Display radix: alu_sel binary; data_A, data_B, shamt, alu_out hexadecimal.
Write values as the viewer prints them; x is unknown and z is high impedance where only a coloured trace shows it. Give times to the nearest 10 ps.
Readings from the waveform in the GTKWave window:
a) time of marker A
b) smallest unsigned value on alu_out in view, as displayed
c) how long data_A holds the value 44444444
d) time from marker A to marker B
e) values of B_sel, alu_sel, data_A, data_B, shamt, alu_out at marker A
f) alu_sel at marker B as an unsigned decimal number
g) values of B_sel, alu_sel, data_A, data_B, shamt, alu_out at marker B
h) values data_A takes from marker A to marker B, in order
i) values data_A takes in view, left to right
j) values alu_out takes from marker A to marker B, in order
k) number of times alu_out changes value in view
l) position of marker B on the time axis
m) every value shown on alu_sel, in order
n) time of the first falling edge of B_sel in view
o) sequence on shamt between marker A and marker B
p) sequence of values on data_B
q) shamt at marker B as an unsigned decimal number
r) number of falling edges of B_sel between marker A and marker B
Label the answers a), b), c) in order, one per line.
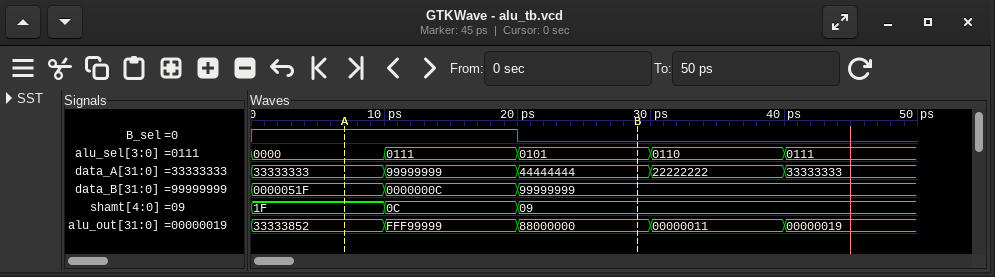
a) 10 ps
b) 00000011
c) 10 ps
d) 20 ps
e) B_sel=1, alu_sel=0000, data_A=33333333, data_B=0000051F, shamt=1F, alu_out=33333852
f) 5
g) B_sel=0, alu_sel=0101, data_A=44444444, data_B=99999999, shamt=09, alu_out=88000000
h) 33333333, 99999999, 44444444
i) 33333333, 99999999, 44444444, 22222222, 33333333
j) 33333852, FFF99999, 88000000
k) 4
l) 30 ps
m) 0000, 0111, 0101, 0110, 0111
n) 20 ps
o) 1F, 0C, 09
p) 0000051F, 0000000C, 99999999
q) 9
r) 1
